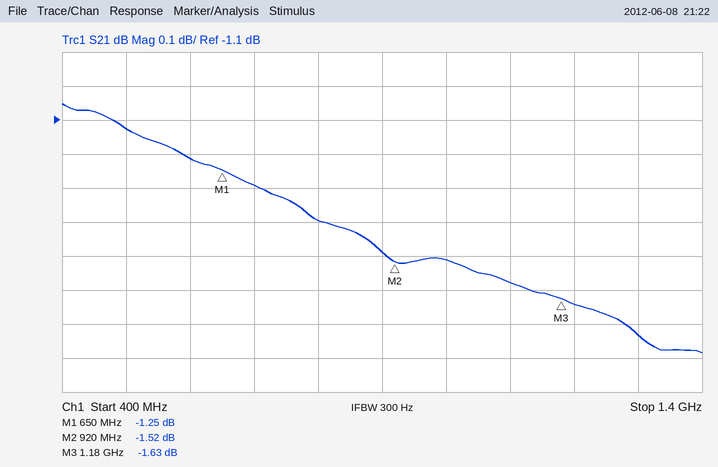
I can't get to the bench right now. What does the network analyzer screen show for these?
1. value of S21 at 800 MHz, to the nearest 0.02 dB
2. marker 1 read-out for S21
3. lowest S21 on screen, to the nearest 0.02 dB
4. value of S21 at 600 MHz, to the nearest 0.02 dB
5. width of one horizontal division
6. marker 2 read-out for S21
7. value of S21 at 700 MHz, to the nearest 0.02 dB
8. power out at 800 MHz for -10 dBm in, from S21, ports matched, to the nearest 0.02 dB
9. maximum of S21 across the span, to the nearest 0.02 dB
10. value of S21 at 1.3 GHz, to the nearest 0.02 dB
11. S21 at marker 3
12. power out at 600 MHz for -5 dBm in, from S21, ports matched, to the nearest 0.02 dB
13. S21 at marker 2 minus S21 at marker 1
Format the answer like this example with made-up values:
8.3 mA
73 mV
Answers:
-1.40 dB
-1.25 dB
-1.78 dB
-1.22 dB
100 MHz
-1.52 dB
-1.30 dB
-11.40 dBm
-1.06 dB
-1.74 dB
-1.63 dB
-6.22 dBm
-0.27 dB
